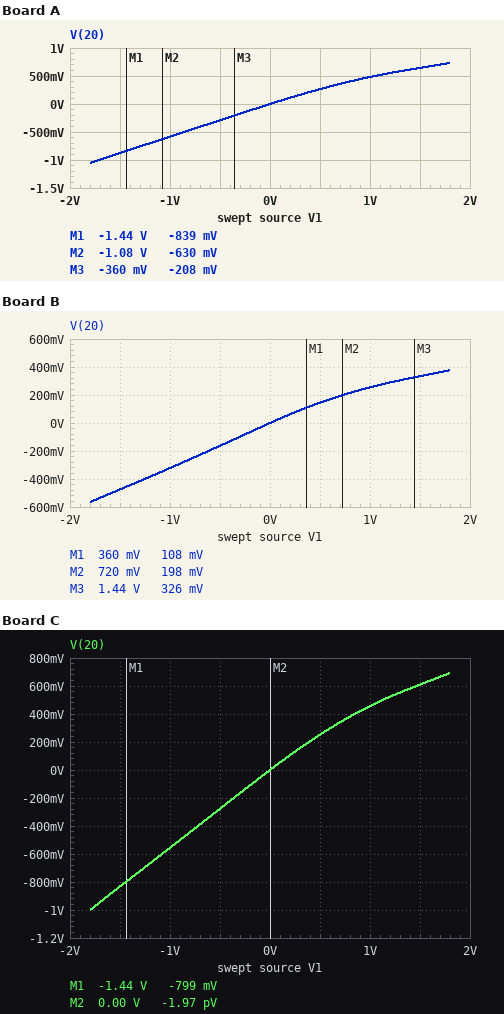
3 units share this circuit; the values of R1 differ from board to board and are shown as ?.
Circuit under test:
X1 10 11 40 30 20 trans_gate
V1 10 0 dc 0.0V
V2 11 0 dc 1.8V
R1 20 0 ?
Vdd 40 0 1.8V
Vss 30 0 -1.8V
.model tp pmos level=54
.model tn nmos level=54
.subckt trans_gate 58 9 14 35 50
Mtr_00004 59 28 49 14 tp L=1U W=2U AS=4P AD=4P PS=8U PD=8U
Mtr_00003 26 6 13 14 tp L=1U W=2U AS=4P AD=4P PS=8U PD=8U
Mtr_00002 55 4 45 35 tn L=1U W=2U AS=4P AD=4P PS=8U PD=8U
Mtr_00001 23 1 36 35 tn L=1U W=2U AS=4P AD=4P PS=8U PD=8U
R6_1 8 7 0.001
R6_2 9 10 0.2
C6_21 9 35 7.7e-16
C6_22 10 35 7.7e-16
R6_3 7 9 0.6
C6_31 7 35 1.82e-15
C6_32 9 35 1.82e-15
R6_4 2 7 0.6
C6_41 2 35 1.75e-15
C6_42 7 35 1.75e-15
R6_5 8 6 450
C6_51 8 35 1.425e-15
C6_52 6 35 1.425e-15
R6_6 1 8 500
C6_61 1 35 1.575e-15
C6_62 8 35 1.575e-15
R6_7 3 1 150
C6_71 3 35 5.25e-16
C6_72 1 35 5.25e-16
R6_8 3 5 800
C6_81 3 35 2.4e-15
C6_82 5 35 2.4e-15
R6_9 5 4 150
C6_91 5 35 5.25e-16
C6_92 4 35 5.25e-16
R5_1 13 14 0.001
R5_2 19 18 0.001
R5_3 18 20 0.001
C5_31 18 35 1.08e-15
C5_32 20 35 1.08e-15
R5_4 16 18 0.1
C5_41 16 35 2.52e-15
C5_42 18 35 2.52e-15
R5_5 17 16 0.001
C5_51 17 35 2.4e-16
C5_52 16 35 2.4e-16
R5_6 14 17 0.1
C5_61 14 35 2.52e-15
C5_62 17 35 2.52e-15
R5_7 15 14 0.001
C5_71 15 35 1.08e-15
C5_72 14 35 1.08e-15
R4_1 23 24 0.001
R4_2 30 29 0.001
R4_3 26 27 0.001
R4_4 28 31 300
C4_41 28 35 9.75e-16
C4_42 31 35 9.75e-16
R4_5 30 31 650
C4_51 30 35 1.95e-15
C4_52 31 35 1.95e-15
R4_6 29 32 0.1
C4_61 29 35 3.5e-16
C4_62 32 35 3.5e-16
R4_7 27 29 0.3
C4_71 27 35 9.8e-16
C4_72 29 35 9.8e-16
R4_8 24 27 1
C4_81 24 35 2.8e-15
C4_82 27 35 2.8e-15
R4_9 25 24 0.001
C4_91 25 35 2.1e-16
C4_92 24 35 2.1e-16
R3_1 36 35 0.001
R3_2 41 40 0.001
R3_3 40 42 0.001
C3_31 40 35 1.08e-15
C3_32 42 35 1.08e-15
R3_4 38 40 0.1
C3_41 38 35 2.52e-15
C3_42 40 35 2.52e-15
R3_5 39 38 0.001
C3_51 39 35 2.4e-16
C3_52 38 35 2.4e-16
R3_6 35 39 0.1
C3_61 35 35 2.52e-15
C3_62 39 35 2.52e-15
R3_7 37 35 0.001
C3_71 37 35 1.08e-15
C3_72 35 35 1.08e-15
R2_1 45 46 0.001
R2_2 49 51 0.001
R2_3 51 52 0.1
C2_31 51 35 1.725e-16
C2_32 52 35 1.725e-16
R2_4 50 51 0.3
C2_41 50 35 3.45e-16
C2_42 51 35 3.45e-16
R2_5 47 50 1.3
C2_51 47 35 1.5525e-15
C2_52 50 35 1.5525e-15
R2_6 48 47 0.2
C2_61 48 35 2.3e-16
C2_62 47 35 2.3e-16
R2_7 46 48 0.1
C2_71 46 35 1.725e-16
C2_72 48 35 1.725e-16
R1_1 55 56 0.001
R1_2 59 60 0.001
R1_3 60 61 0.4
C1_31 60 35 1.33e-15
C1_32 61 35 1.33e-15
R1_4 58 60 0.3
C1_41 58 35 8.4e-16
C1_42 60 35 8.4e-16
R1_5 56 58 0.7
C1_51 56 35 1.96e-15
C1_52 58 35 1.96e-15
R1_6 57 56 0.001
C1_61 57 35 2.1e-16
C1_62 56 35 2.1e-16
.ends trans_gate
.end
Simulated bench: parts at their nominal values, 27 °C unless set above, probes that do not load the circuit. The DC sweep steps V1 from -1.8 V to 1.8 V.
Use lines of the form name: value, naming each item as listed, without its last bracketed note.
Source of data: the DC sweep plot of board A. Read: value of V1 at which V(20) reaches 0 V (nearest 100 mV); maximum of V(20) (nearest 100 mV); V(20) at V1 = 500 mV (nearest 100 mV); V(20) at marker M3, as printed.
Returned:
value of V1 at which V(20) reaches 0 V: 0 V
maximum of V(20): 700 mV
V(20) at V1 = 500 mV: 300 mV
V(20) at marker M3, as printed: -208 mV
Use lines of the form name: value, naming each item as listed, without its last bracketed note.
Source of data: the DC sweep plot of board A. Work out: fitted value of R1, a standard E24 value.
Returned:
fitted value of R1, a standard E24 value: 910 Ω
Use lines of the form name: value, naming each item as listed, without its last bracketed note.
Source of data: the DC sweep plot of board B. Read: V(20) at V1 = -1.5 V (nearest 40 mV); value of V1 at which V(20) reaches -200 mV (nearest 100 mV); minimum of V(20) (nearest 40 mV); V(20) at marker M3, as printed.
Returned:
V(20) at V1 = -1.5 V: -480 mV
value of V1 at which V(20) reaches -200 mV: -600 mV
minimum of V(20): -560 mV
V(20) at marker M3, as printed: 326 mV
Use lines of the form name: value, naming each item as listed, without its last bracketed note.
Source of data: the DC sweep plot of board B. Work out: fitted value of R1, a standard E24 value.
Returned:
fitted value of R1, a standard E24 value: 330 Ω
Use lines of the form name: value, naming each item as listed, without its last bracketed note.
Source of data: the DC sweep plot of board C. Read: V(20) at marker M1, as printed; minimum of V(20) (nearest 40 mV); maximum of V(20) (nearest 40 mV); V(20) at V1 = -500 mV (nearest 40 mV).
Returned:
V(20) at marker M1, as printed: -799 mV
minimum of V(20): -1.00 V
maximum of V(20): 680 mV
V(20) at V1 = -500 mV: -280 mV
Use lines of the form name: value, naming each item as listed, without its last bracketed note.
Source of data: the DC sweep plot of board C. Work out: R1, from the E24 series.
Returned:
R1, from the E24 series: 820 Ω
